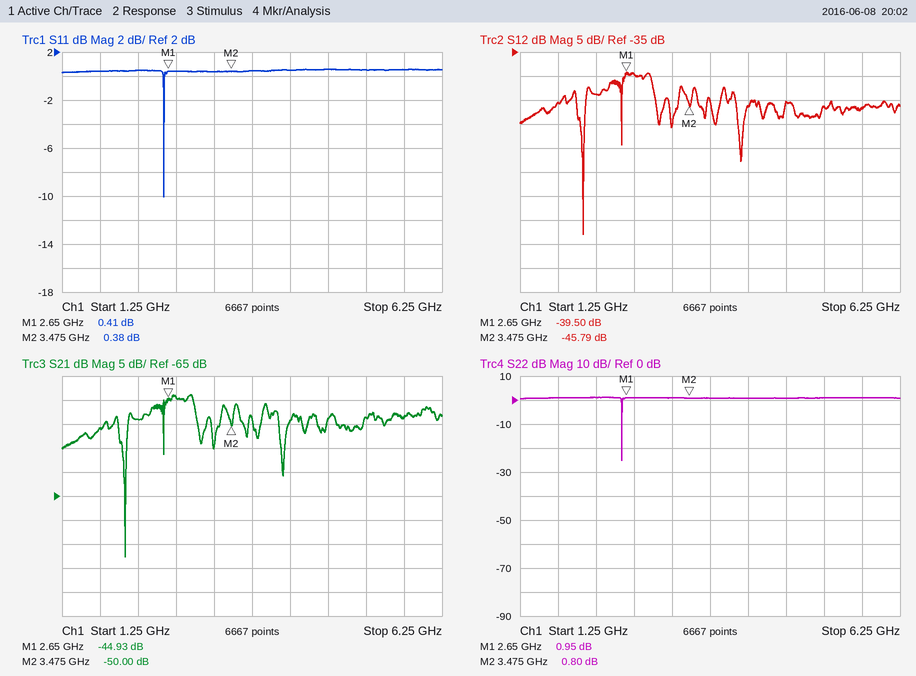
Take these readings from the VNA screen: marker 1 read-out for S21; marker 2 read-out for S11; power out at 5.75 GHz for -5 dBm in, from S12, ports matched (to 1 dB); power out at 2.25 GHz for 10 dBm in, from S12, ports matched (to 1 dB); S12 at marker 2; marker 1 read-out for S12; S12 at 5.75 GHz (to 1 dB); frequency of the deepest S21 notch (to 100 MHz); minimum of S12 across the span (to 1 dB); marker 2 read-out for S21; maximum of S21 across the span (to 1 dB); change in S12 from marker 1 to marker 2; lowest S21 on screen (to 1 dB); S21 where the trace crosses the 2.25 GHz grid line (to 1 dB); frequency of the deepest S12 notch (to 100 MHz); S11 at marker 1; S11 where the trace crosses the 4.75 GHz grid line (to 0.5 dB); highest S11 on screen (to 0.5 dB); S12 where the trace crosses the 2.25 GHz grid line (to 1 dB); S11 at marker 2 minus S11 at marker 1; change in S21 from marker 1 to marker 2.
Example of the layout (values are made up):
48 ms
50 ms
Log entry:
-44.93 dB
0.38 dB
-52 dBm
-34 dBm
-45.79 dB
-39.50 dB
-47 dB
2.1 GHz
-73 dB
-50.00 dB
-44 dB
-6.29 dB
-78 dB
-49 dB
2.1 GHz
0.41 dB
0.5 dB
0.5 dB
-44 dB
-0.03 dB
-5.07 dB
